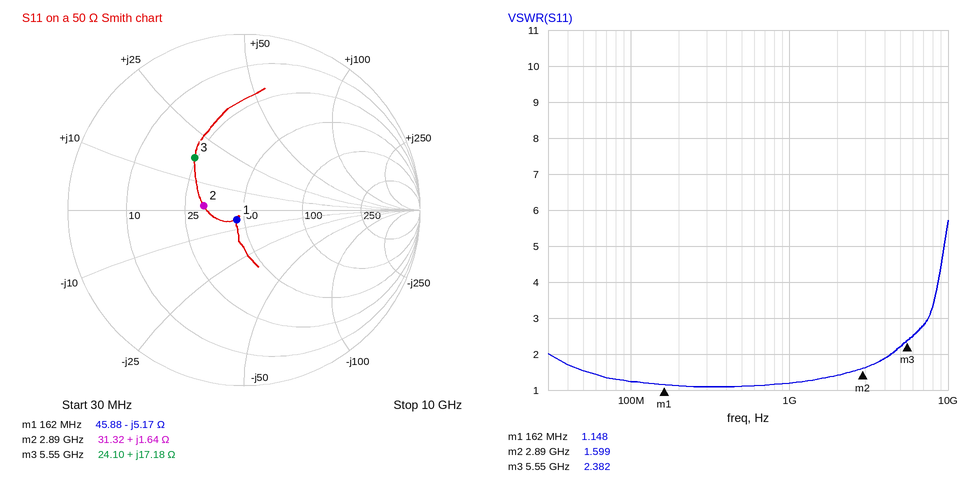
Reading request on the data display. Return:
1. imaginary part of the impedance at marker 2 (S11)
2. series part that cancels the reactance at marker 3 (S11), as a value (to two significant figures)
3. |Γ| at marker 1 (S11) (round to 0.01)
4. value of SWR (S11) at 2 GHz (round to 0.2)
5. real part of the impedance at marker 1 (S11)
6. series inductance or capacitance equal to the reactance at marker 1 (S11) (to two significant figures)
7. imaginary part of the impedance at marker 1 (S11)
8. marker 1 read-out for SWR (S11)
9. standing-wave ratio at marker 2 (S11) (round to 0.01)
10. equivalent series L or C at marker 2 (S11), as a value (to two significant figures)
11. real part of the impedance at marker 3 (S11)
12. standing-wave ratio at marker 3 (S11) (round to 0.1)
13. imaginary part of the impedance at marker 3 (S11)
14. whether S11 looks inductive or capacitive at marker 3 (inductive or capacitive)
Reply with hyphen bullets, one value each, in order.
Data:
- +1.64 Ω
- 1.7 pF
- 0.07
- 1.4
- 45.88 Ω
- 190 pF
- -5.17 Ω
- 1.148
- 1.60
- 90 pH
- 24.10 Ω
- 2.4
- +17.18 Ω
- inductive
